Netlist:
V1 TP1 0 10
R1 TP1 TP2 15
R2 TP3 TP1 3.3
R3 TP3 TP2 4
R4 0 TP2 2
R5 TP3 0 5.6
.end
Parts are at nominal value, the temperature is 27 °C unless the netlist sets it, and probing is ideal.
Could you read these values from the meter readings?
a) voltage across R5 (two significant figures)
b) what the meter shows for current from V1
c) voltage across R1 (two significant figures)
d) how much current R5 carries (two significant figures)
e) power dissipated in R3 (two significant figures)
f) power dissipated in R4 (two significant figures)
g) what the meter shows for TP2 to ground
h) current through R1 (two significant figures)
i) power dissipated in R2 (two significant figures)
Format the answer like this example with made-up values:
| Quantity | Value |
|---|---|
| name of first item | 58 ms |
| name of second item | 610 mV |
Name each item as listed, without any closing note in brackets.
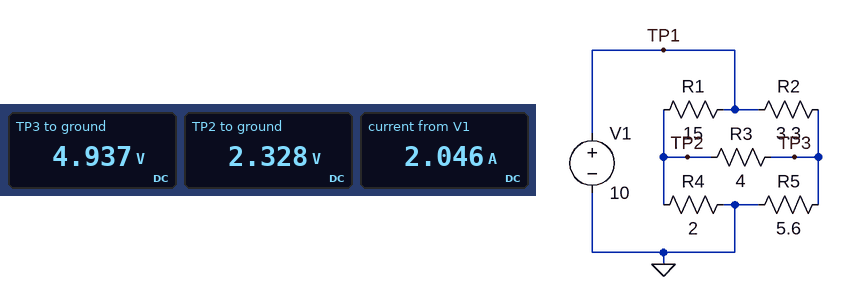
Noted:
| Quantity | Value |
|---|---|
| voltage across R5 | 4.9 V |
| what the meter shows for current from V1 | 2.046 A |
| voltage across R1 | 7.7 V |
| how much current R5 carries | 880 mA |
| power dissipated in R3 | 1.7 W |
| power dissipated in R4 | 2.7 W |
| what the meter shows for TP2 to ground | 2.328 V |
| current through R1 | 510 mA |
| power dissipated in R2 | 7.8 W |
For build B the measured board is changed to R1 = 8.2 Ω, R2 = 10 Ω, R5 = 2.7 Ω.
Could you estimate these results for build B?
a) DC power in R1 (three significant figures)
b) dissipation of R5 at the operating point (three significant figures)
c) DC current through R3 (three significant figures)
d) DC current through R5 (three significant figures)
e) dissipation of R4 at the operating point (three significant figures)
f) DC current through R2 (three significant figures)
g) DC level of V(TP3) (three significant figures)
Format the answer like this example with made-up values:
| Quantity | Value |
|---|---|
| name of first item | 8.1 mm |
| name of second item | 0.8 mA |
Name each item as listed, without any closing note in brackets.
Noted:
| Quantity | Value |
|---|---|
| DC power in R1 | 7.81 W |
| dissipation of R5 at the operating point | 1.60 W |
| DC current through R3 | 21.4 mA |
| DC current through R5 | 771 mA |
| dissipation of R4 at the operating point | 1.99 W |
| DC current through R2 | 792 mA |
| DC level of V(TP3) | 2.08 V |
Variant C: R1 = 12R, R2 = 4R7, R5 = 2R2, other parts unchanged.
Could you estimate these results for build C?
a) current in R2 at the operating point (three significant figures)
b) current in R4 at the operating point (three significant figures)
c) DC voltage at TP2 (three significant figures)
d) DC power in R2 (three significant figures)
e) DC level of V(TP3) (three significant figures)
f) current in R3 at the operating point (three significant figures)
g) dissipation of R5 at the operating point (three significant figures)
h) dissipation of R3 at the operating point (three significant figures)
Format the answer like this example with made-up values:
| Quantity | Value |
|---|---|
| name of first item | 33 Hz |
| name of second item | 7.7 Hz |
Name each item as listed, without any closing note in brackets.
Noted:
| Quantity | Value |
|---|---|
| current in R2 at the operating point | 1.53 A |
| current in R4 at the operating point | 923 mA |
| DC voltage at TP2 | 1.85 V |
| DC power in R2 | 11.0 W |
| DC level of V(TP3) | 2.82 V |
| current in R3 at the operating point | 244 mA |
| dissipation of R5 at the operating point | 3.62 W |
| dissipation of R3 at the operating point | 238 mW |
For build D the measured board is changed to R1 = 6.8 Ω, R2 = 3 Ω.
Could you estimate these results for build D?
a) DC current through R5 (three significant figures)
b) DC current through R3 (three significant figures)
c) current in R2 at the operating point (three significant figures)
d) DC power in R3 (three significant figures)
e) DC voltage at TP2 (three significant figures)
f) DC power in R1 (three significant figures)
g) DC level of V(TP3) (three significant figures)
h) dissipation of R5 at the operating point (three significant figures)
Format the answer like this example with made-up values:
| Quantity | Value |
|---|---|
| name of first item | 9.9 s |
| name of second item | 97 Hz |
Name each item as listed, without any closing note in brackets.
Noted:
| Quantity | Value |
|---|---|
| DC current through R5 | 966 mA |
| DC current through R3 | 565 mA |
| current in R2 at the operating point | 1.53 A |
| DC power in R3 | 1.28 W |
| DC voltage at TP2 | 3.15 V |
| DC power in R1 | 6.91 W |
| DC level of V(TP3) | 5.41 V |
| dissipation of R5 at the operating point | 5.22 W |
